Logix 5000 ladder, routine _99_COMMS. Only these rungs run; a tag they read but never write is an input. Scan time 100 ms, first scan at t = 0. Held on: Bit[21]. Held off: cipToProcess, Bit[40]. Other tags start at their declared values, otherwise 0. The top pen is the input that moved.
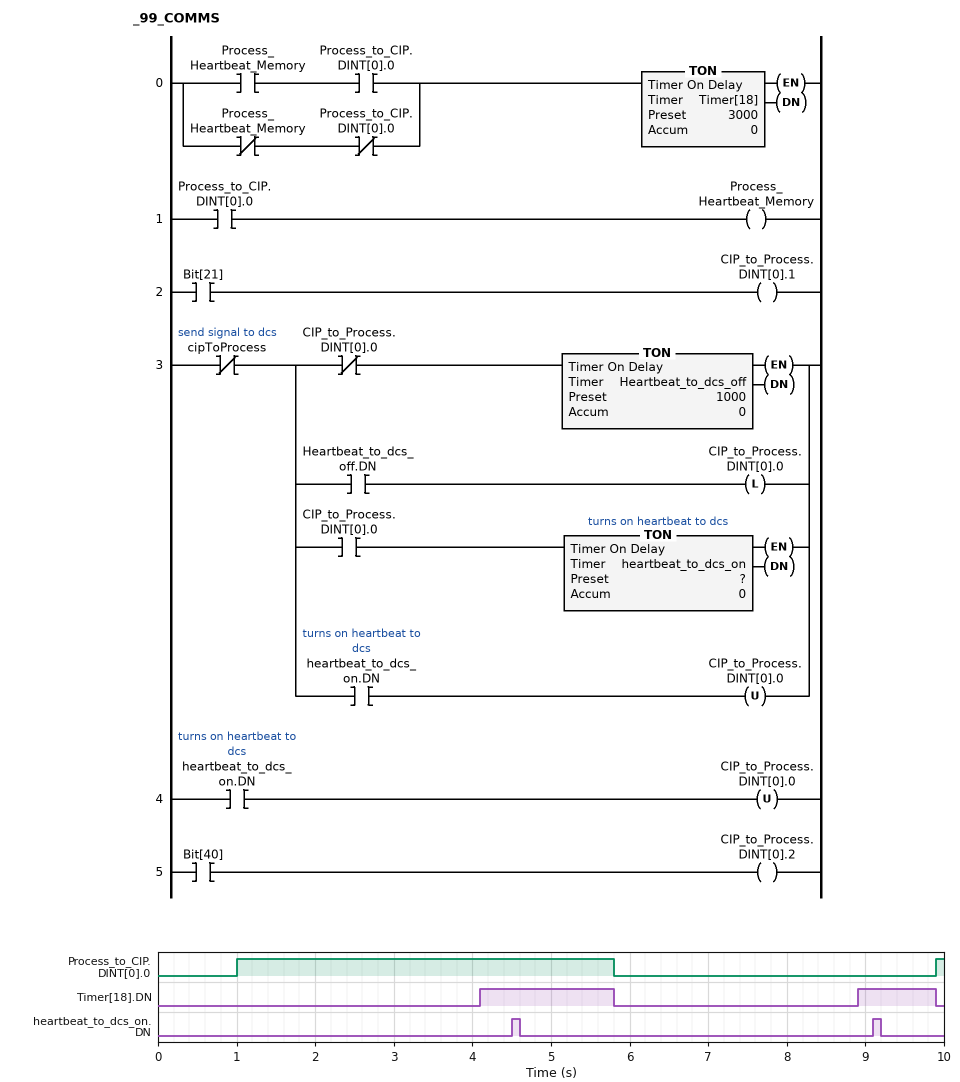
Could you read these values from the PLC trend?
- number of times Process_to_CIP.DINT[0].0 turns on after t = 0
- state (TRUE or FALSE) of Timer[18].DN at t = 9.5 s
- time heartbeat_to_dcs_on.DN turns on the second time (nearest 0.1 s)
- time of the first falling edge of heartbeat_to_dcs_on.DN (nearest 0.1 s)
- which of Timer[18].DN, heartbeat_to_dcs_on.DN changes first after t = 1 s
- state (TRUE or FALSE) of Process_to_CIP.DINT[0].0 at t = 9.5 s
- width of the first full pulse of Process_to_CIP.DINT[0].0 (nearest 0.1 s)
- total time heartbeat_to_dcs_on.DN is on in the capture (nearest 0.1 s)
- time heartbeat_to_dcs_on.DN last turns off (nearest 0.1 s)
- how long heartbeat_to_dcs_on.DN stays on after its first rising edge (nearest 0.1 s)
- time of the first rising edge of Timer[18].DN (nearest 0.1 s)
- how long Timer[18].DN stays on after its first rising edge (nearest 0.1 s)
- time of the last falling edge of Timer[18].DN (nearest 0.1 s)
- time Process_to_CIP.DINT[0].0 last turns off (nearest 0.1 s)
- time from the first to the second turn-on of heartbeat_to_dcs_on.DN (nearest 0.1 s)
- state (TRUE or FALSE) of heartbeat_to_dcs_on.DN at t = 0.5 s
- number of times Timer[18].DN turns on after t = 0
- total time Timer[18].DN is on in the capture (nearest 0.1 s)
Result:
2
TRUE
9.1 s
4.6 s
Timer[18].DN
FALSE
4.8 s
0.2 s
9.2 s
0.1 s
4.1 s
1.7 s
9.9 s
5.8 s
4.6 s
FALSE
2
2.7 s
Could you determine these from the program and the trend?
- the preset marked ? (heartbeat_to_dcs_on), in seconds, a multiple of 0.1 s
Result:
3.5 s
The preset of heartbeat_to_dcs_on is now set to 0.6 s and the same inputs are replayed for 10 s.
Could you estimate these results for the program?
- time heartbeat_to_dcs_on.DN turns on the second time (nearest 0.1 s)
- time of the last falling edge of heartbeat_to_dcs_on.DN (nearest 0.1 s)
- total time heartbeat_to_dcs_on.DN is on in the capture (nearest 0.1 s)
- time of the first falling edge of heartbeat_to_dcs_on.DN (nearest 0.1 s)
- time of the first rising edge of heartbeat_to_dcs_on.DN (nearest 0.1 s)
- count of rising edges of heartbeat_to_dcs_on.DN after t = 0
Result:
3.3 s
8.5 s
0.5 s
1.7 s
1.6 s
5
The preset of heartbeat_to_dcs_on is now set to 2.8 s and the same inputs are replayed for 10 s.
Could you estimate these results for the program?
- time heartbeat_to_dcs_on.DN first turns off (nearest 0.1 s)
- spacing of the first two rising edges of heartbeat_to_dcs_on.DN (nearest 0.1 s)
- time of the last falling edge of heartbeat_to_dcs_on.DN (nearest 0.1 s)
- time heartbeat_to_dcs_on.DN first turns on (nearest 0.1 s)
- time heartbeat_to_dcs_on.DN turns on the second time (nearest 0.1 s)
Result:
3.9 s
3.9 s
7.8 s
3.8 s
7.7 s
